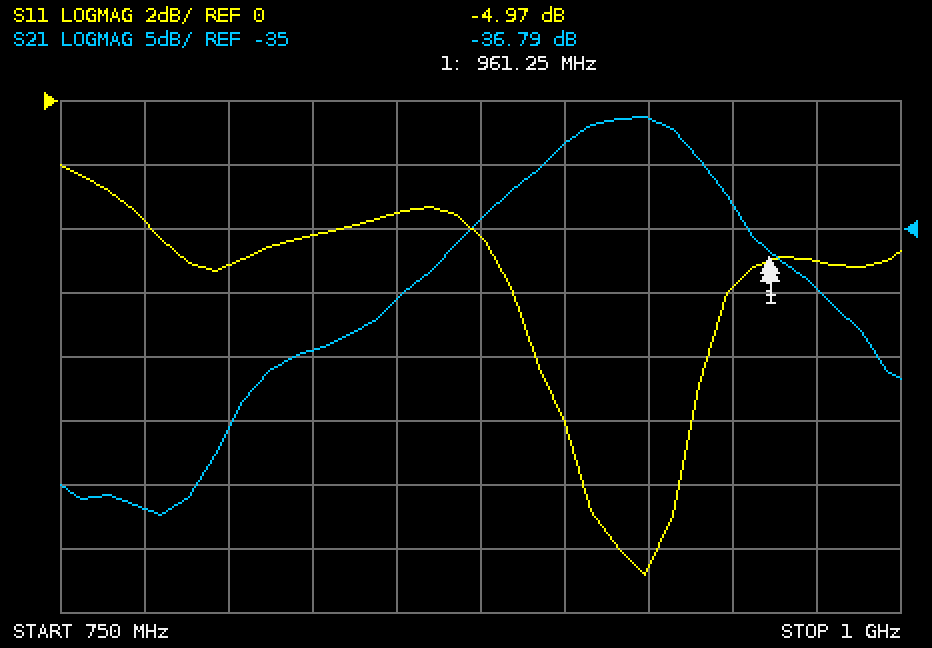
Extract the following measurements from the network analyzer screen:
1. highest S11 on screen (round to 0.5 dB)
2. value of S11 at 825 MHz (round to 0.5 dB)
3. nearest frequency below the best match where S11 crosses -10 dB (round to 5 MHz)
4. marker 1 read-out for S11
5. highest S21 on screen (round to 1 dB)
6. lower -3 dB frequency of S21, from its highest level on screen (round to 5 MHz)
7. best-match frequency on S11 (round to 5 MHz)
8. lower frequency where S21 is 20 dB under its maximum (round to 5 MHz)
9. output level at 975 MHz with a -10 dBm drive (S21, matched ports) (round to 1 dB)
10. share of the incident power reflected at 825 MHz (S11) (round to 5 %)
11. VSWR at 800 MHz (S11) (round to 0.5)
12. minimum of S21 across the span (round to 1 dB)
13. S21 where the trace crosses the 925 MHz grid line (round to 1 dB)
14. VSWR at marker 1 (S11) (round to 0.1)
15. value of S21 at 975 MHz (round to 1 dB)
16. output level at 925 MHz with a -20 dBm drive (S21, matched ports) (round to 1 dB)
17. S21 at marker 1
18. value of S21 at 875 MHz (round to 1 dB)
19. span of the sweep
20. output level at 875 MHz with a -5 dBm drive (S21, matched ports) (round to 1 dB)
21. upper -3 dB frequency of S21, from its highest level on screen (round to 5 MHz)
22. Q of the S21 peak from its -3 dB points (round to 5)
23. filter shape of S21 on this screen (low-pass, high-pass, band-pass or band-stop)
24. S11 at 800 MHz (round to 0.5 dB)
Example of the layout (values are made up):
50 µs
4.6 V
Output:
-2.0 dB
-4.0 dB
900 MHz
-4.97 dB
-26 dB
895 MHz
925 MHz
810 MHz
-50 dBm
40 %
3.5
-57 dB
-26 dB
3.6
-40 dB
-46 dBm
-36.79 dB
-34 dB
250 MHz
-39 dBm
940 MHz
20
band-pass
-5.0 dB
